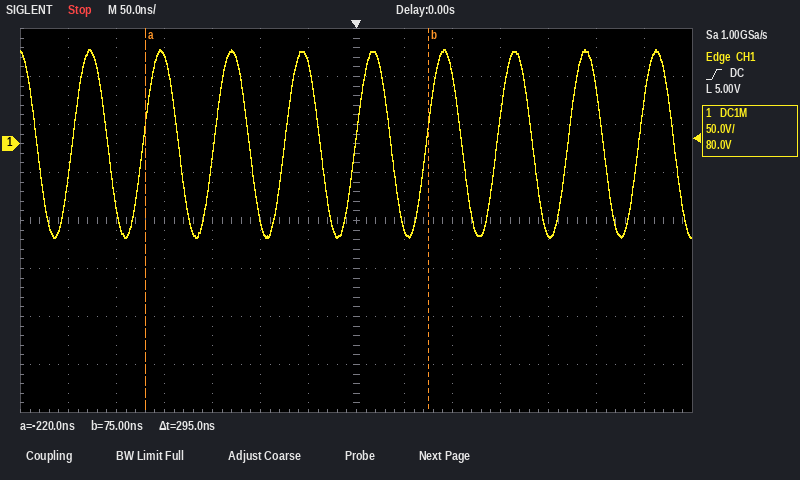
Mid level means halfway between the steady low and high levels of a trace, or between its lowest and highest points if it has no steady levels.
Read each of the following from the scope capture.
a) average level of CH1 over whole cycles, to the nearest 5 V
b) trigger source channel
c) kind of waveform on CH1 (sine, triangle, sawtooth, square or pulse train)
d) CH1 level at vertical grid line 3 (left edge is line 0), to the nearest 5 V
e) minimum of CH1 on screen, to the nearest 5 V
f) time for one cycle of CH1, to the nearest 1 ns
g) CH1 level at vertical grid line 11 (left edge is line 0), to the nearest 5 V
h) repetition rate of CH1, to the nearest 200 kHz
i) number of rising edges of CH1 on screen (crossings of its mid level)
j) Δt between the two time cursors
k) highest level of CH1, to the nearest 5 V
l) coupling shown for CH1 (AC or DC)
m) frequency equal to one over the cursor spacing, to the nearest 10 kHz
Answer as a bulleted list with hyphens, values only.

- 0 V
- CH1
- sine
- 90 V
- -100 V
- 74 ns
- -95 V
- 13.6 MHz
- 9
- 295 ns
- 100 V
- DC
- 3.39 MHz
